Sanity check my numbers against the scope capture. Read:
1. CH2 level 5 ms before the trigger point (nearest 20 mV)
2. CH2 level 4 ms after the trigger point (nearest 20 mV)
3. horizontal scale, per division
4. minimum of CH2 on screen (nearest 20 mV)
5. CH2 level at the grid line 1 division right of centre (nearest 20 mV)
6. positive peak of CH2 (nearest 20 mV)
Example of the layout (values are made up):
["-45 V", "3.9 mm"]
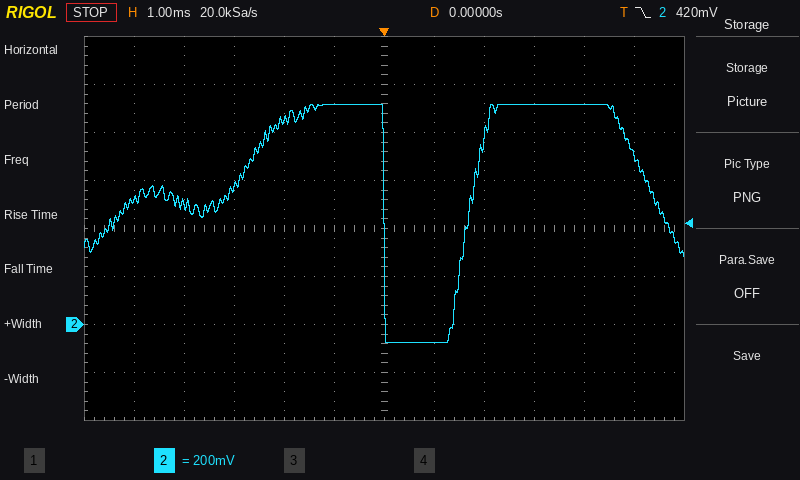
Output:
["520 mV", "920 mV", "1 ms", "-80 mV", "-80 mV", "920 mV"]
